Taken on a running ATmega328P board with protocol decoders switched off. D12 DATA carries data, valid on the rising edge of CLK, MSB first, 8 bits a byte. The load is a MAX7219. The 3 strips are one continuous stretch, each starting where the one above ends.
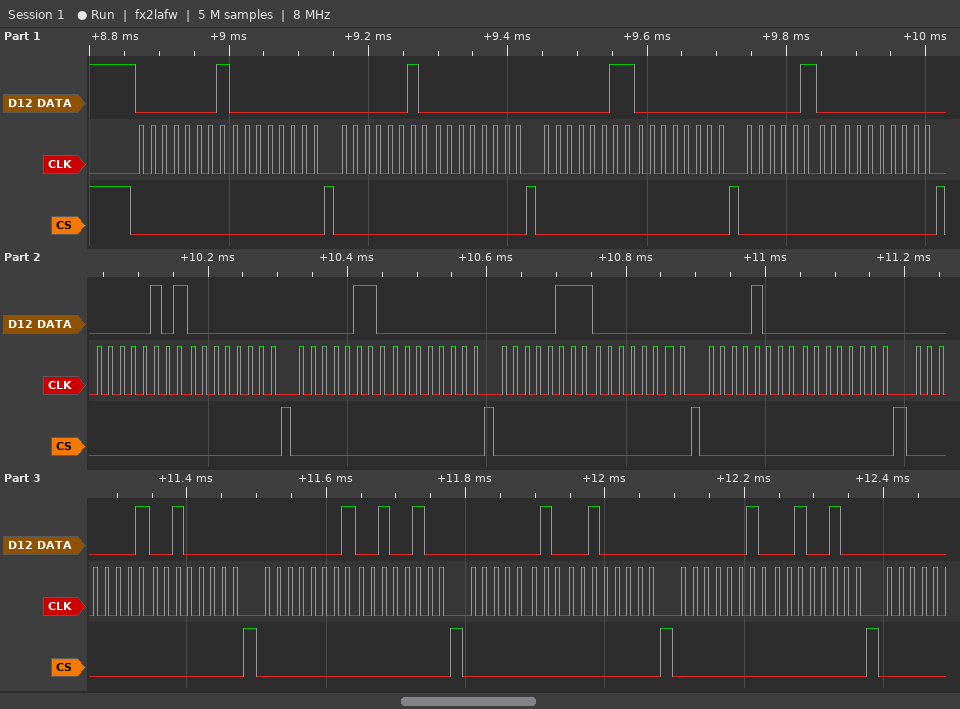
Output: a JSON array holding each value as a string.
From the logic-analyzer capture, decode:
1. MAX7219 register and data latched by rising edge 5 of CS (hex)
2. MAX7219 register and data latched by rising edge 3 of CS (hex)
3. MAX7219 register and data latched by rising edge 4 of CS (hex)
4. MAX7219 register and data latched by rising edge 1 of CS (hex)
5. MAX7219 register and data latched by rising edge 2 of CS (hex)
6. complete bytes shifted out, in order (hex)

["register 0x5, data 0x00", "register 0x3, data 0x00", "register 0x4, data 0x00", "register 0x1, data 0x00", "register 0x2, data 0x00", "01 00 02 00 03 00 04 00 05 00 06 00 07 00 08 00 01 20 01 24 02 20 02 24"]
